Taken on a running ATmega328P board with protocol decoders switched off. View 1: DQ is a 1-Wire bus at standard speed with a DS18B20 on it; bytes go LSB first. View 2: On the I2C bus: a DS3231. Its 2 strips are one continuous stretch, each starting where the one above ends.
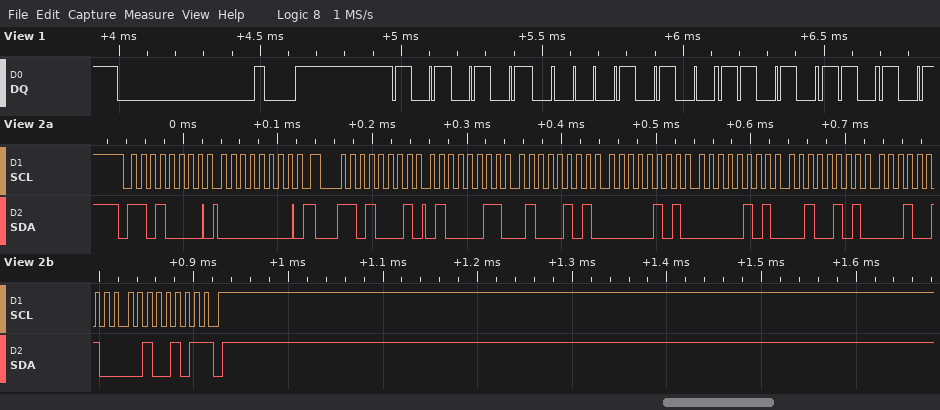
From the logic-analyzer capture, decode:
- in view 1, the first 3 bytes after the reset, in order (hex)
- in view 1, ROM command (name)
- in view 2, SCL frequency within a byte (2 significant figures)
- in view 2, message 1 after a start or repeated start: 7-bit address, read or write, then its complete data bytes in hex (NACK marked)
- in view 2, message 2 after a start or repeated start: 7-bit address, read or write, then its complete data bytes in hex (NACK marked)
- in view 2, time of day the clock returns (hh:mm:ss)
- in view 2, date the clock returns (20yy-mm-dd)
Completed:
55 28 6B
Match ROM
100 kHz
0x68 write: 00
0x68 read: 43 45 05 05 25 12 25 NACK
05:45:43
2025-12-25
